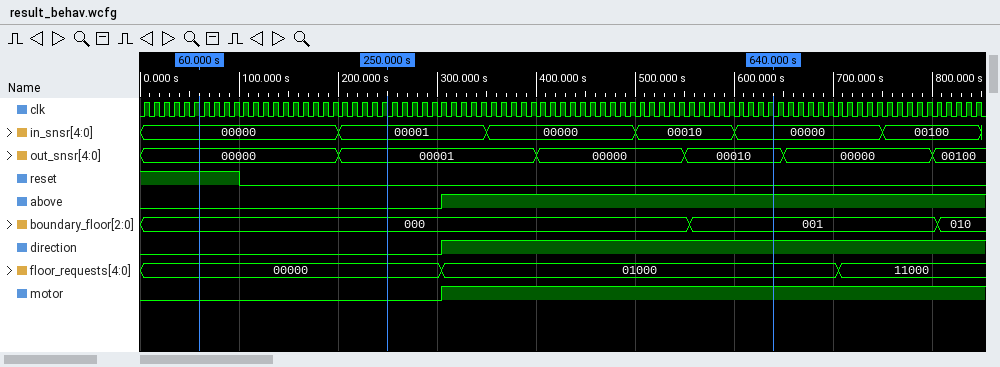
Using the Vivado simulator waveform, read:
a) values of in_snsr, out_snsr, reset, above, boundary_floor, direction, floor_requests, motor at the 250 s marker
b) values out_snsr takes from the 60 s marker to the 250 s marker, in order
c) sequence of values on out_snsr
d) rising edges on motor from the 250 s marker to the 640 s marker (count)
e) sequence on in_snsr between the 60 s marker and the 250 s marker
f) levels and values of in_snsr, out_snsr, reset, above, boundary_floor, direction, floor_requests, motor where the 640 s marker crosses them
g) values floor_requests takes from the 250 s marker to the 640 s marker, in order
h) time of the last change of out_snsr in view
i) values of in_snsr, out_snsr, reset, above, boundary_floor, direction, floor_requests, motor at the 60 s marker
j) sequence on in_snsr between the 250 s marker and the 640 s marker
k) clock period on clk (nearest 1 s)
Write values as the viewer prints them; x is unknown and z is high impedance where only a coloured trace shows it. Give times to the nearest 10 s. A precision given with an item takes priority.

in_snsr=00001, out_snsr=00001, reset=0, above=0, boundary_floor=000, direction=0, floor_requests=00000, motor=0
00000, 00001
00000, 00001, 00000, 00010, 00000, 00100
1
00000, 00001
in_snsr=00000, out_snsr=00010, reset=0, above=1, boundary_floor=001, direction=1, floor_requests=01000, motor=1
00000, 01000
800 s
in_snsr=00000, out_snsr=00000, reset=1, above=0, boundary_floor=000, direction=0, floor_requests=00000, motor=0
00001, 00000, 00010, 00000
10 s
